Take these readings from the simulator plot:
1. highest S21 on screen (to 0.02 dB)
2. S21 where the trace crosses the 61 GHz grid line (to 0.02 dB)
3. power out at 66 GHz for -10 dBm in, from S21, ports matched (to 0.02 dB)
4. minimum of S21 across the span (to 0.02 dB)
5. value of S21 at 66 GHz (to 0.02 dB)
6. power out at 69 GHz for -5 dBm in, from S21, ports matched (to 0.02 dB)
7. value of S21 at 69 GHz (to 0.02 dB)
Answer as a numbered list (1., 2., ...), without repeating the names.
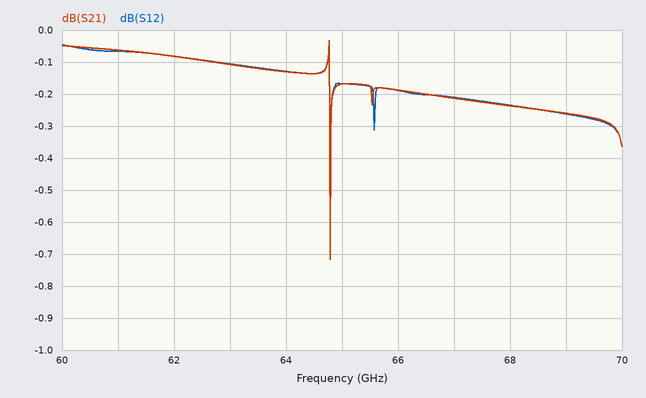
1. -0.04 dB
2. -0.06 dB
3. -10.18 dBm
4. -0.72 dB
5. -0.18 dB
6. -5.26 dBm
7. -0.26 dB
